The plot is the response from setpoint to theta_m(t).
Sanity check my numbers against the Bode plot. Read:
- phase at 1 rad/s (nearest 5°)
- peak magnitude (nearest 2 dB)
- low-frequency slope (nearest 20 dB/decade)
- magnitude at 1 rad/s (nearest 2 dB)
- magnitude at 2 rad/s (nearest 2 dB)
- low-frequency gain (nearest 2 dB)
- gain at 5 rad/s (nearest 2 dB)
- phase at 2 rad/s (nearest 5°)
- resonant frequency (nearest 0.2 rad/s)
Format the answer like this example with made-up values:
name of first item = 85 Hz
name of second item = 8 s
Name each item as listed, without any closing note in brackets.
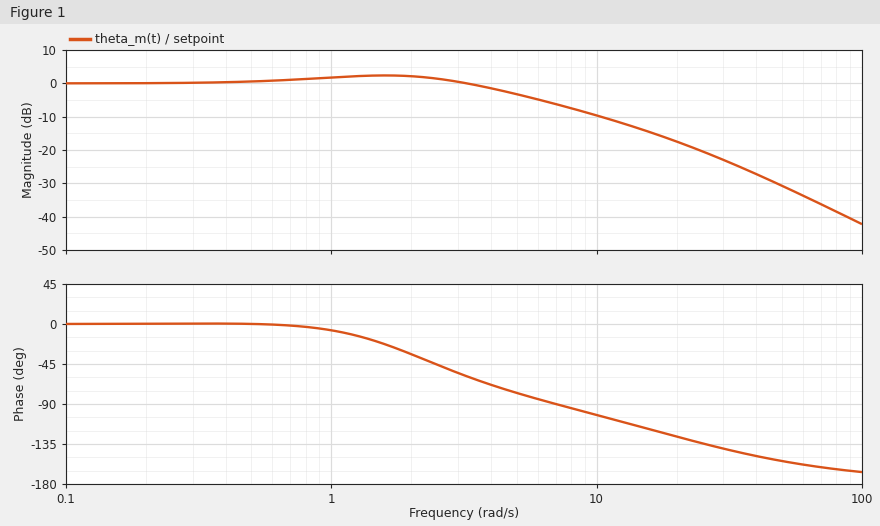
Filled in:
phase at 1 rad/s = -5°
peak magnitude = 2 dB
low-frequency slope = 0 dB/decade
magnitude at 1 rad/s = 2 dB
magnitude at 2 rad/s = 2 dB
low-frequency gain = 0 dB
gain at 5 rad/s = -4 dB
phase at 2 rad/s = -35°
resonant frequency = 1.6 rad/s
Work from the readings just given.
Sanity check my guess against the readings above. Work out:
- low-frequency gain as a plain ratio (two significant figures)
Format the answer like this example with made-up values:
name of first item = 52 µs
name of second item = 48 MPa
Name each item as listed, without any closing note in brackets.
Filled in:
low-frequency gain as a plain ratio = 1.0
